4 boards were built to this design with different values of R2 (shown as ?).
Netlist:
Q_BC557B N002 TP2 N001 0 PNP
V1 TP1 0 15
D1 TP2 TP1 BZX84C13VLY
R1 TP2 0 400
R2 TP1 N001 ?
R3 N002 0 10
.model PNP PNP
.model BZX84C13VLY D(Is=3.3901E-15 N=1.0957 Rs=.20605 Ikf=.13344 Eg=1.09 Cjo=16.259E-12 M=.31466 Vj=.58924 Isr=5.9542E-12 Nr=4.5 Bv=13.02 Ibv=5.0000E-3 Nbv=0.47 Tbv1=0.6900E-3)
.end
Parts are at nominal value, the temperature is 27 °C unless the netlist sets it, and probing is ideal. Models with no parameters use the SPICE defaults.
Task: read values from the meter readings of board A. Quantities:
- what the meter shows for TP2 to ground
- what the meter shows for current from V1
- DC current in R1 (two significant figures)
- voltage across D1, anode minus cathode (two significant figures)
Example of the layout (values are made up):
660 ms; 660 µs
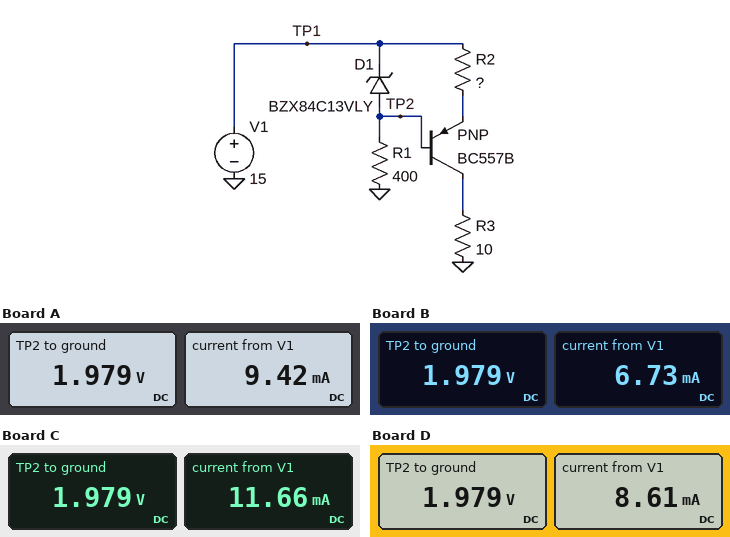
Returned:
1.979 V; 9.42 mA; 4.9 mA; -13 V
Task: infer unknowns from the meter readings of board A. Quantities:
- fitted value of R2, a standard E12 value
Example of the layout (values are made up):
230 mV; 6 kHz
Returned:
2.7 kΩ
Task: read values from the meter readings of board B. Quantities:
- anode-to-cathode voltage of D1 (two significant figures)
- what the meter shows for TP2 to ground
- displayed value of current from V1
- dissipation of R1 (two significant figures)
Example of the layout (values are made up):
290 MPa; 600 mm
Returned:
-13 V; 1.979 V; 6.73 mA; 9.8 mW
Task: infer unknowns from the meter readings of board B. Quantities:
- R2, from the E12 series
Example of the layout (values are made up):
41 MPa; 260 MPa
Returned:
6.8 kΩ
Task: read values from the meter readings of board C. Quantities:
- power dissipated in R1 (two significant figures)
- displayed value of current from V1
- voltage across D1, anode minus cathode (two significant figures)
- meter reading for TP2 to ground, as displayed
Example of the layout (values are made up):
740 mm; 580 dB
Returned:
9.8 mW; 11.66 mA; -13 V; 1.979 V
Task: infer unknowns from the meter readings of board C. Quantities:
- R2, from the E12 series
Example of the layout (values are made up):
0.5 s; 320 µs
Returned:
1.8 kΩ
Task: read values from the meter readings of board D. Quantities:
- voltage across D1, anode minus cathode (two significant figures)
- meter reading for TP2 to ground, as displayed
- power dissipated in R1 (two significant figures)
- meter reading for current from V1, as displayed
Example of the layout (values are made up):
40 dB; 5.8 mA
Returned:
-13 V; 1.979 V; 9.8 mW; 8.61 mA
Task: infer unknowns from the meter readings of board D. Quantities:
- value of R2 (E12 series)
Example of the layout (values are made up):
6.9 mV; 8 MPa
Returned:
3.3 kΩ
